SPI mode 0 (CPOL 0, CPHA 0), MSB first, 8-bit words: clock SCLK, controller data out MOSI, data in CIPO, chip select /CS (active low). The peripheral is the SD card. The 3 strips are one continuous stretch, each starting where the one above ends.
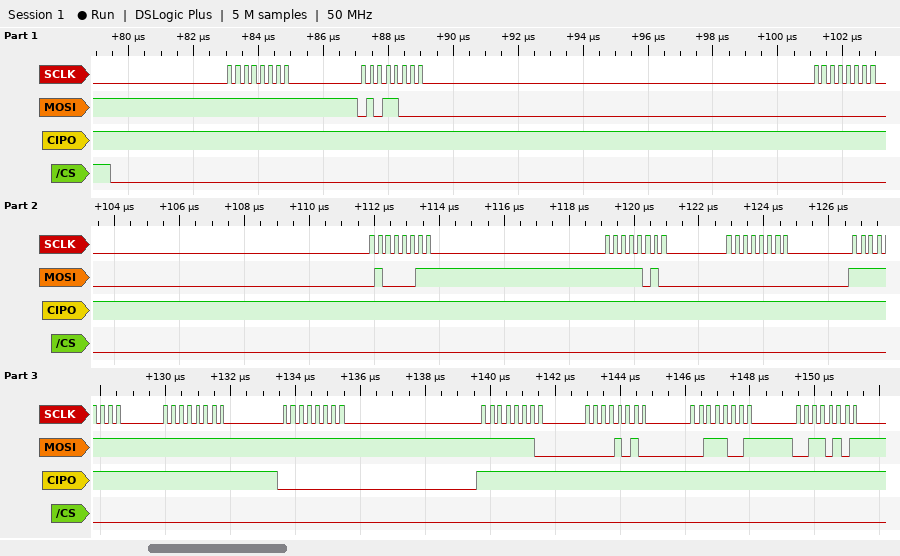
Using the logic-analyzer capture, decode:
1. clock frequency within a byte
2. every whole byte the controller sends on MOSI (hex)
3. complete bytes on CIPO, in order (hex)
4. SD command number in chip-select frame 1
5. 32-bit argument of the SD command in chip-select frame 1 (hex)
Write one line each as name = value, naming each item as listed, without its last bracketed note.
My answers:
clock frequency within a byte = 4 MHz
every whole byte the controller sends on MOSI = FF 58 00 43 FA 00 FF FF FF FE 0A 39 35
complete bytes on CIPO, in order = FF FF FF FF FF FF FF FF 00 FF FF FF FF
SD command number in chip-select frame 1 = CMD24
32-bit argument of the SD command in chip-select frame 1 = 0x0043FA00
